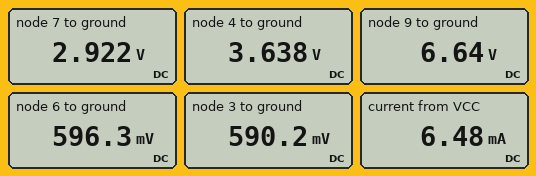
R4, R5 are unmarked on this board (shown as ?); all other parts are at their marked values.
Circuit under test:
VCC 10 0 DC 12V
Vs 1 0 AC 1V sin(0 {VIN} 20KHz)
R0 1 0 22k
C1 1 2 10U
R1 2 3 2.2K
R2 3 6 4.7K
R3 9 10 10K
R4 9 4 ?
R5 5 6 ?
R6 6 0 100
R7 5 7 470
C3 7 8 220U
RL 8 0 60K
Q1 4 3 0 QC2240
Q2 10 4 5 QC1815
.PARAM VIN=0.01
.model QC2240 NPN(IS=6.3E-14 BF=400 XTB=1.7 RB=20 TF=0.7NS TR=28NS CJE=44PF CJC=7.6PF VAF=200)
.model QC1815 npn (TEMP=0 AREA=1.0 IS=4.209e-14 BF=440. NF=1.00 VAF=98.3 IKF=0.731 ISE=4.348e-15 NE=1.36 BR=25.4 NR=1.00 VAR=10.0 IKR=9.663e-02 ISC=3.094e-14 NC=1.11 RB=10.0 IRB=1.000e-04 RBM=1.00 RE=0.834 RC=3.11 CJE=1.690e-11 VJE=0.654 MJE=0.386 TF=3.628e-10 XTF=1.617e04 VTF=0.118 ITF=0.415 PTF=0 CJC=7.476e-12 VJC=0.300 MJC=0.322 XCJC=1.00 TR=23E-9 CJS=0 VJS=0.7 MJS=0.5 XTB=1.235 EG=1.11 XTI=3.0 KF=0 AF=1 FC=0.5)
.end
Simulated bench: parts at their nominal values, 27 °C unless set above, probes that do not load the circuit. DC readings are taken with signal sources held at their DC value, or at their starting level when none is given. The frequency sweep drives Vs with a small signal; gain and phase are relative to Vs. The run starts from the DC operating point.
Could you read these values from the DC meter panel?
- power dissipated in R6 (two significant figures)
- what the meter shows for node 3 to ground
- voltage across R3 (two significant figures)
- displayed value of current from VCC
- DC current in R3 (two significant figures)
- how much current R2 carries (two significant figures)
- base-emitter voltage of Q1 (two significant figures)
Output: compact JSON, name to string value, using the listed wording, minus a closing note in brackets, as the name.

{"power dissipated in R6": "3.6 mW", "what the meter shows for node 3 to ground": "590.2 mV", "voltage across R3": "5.4 V", "displayed value of current from VCC": "6.48 mA", "DC current in R3": "540 µA", "how much current R2 carries": "1.3 µA", "base-emitter voltage of Q1": "590 mV"}
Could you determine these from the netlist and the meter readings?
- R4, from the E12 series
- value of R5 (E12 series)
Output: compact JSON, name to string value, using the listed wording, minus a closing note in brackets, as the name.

{"R4, from the E12 series": "5.6 kΩ", "value of R5": "390 Ω"}
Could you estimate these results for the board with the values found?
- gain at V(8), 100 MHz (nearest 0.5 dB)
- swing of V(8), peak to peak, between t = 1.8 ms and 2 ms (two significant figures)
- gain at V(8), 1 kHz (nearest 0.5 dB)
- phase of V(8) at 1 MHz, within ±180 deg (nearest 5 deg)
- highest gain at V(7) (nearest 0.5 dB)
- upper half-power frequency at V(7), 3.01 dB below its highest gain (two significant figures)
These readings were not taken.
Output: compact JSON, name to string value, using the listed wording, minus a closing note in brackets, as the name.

{"gain at V(8), 100 MHz": "-29.5 dB", "swing of V(8), peak to peak, between t = 1.8 ms and 2 ms": "200 mV", "gain at V(8), 1 kHz": "20.0 dB", "phase of V(8) at 1 MHz, within ±180 deg": "145 deg", "highest gain at V(7)": "20.0 dB", "upper half-power frequency at V(7), 3.01 dB below its highest gain": "1.5 MHz"}
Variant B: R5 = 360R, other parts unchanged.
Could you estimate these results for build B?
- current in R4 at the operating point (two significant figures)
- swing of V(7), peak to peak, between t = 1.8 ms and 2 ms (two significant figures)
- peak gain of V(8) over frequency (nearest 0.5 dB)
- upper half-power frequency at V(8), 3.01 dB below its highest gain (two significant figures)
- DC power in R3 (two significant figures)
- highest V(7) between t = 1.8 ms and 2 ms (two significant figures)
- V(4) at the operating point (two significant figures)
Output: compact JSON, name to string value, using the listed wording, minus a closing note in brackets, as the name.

{"current in R4 at the operating point": "550 µA", "swing of V(7), peak to peak, between t = 1.8 ms and 2 ms": "190 mV", "peak gain of V(8) over frequency": "19.5 dB", "upper half-power frequency at V(8), 3.01 dB below its highest gain": "1.6 MHz", "DC power in R3": "3.0 mW", "highest V(7) between t = 1.8 ms and 2 ms": "2.8 V", "V(4) at the operating point": "3.5 V"}
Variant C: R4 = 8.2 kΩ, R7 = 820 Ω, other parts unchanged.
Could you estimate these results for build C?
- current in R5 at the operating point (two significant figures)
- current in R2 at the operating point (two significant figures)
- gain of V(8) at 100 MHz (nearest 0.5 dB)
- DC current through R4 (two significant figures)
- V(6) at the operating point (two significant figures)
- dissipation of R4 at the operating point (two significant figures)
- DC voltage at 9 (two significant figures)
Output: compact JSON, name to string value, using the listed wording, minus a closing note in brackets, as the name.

{"current in R5 at the operating point": "5.9 mA", "current in R2 at the operating point": "1.1 µA", "gain of V(8) at 100 MHz": "-30.5 dB", "DC current through R4": "460 µA", "V(6) at the operating point": "590 mV", "dissipation of R4 at the operating point": "1.7 mW", "DC voltage at 9": "7.4 V"}
